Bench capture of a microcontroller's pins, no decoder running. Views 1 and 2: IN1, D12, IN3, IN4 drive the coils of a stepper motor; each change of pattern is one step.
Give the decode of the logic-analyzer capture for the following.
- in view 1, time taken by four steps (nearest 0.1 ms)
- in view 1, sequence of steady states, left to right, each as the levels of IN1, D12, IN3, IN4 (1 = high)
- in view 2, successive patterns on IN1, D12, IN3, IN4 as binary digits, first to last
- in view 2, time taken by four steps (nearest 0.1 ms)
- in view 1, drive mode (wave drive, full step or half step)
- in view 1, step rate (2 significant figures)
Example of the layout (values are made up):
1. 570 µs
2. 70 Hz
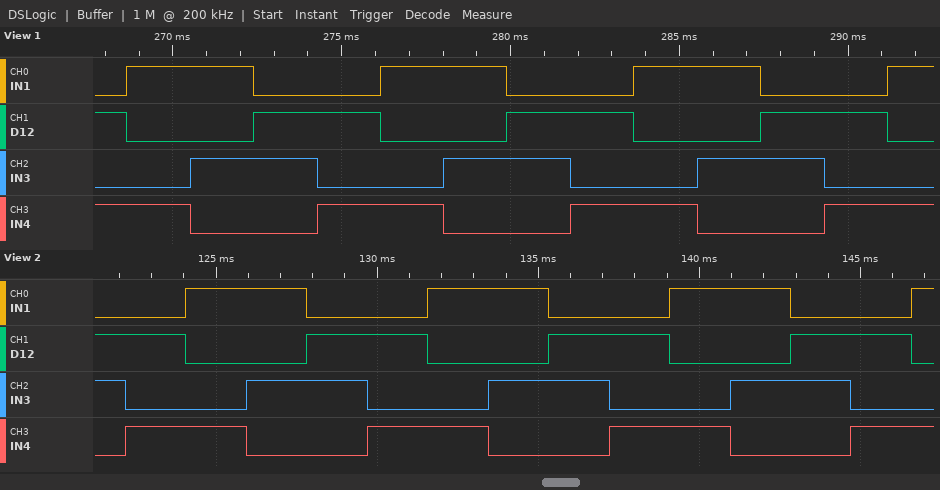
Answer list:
1. 7.5 ms
2. 0101 1001 1010 0110 0101 1001 1010 0110 0101 1001 1010 0110 0101 1001
3. 0110 0101 1001 1010 0110 0101 1001 1010 0110 0101 1001 1010 0110 0101 1001
4. 7.5 ms
5. full step
6. 530 steps/s
